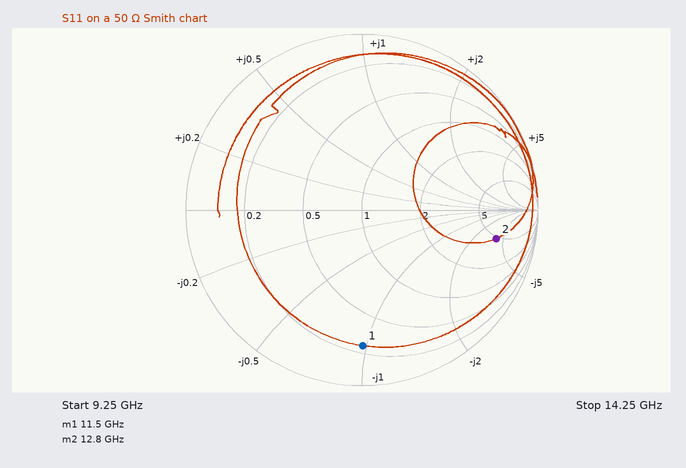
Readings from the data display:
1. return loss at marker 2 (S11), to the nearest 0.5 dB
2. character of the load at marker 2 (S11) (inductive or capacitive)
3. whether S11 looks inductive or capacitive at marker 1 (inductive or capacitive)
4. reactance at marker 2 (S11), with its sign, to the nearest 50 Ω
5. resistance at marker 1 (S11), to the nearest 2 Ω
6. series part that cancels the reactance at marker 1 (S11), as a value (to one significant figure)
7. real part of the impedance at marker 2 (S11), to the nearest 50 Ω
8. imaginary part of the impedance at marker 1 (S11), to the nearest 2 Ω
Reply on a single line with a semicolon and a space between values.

2.0 dB; capacitive; capacitive; -200 Ω; 12 Ω; 700 pH; 250 Ω; -48 Ω
